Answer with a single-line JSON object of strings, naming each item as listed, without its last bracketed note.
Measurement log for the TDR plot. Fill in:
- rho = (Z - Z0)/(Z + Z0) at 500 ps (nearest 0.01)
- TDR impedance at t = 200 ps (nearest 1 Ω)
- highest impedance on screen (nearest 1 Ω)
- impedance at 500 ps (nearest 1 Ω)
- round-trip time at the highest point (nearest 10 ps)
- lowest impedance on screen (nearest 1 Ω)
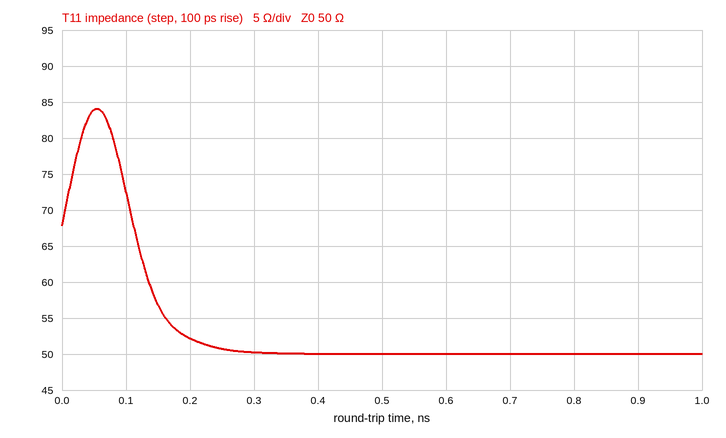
{"rho = (Z - Z0)/(Z + Z0) at 500 ps": "0.00", "TDR impedance at t = 200 ps": "52 Ω", "highest impedance on screen": "84 Ω", "impedance at 500 ps": "50 Ω", "round-trip time at the highest point": "50 ps", "lowest impedance on screen": "50 Ω"}
